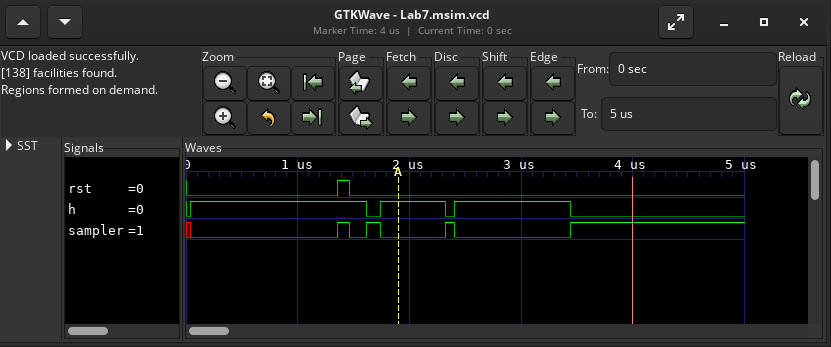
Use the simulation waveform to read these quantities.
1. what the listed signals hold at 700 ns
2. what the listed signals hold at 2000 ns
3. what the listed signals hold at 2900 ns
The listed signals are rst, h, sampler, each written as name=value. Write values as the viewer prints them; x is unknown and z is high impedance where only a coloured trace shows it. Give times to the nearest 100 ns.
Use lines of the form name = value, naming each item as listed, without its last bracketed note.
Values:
what the listed signals hold at 700 ns = rst=0, h=1, sampler=0
what the listed signals hold at 2000 ns = rst=0, h=1, sampler=0
what the listed signals hold at 2900 ns = rst=0, h=1, sampler=0
